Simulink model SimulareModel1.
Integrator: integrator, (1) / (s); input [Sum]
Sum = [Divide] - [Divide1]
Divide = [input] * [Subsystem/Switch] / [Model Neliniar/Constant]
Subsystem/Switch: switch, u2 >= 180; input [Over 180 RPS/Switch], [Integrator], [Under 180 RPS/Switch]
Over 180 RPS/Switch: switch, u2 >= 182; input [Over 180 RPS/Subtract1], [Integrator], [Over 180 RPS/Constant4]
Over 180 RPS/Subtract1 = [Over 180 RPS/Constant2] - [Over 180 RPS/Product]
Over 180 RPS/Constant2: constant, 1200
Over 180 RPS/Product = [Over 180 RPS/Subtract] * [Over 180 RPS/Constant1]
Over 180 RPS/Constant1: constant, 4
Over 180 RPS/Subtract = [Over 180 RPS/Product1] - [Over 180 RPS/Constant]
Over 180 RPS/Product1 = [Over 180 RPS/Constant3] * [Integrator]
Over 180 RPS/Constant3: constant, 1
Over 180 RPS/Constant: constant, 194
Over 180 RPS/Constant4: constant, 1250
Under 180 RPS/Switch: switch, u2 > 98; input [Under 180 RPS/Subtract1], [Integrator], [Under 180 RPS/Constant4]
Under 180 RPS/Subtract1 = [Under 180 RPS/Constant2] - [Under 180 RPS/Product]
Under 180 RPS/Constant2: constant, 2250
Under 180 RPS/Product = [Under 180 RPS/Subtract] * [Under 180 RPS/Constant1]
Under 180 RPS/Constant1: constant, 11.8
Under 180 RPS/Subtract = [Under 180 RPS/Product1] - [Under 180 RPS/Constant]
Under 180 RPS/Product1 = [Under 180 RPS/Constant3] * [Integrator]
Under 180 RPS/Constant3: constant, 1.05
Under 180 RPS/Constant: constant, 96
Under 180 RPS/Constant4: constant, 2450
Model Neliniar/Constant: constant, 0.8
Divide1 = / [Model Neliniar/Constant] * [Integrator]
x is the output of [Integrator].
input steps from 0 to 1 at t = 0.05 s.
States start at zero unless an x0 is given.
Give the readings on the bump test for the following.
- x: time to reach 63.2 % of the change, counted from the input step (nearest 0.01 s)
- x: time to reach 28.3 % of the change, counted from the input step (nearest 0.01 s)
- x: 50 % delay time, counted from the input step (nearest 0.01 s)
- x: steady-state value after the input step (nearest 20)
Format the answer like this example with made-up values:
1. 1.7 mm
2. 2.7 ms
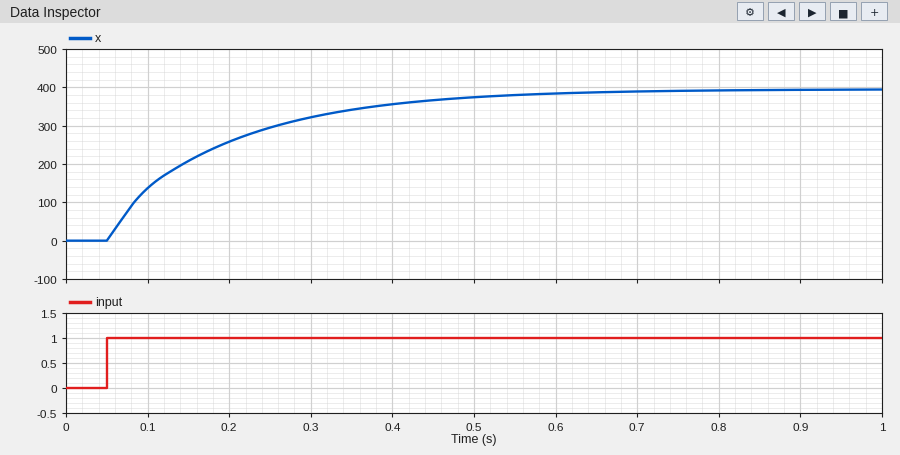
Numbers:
1. 0.14 s
2. 0.04 s
3. 0.09 s
4. 400
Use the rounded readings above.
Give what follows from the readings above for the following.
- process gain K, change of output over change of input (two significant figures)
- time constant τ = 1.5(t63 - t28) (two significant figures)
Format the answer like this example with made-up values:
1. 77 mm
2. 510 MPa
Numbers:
1. 400
2. 0.15 s
